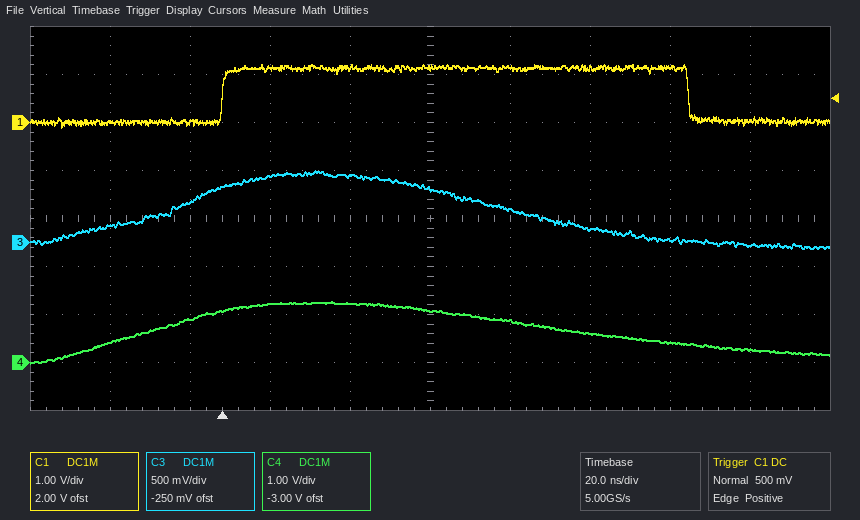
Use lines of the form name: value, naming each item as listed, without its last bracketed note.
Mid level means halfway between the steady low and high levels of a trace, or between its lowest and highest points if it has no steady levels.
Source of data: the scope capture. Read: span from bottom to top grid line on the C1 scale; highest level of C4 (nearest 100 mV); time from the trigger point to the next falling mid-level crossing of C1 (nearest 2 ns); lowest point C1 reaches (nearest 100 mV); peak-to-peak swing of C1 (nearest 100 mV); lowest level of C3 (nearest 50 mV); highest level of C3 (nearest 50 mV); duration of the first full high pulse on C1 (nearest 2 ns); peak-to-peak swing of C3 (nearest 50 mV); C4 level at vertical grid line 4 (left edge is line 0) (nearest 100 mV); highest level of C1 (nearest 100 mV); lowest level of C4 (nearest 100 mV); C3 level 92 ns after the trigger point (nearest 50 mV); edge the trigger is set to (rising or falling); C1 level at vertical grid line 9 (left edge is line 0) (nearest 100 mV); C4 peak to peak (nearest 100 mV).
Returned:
span from bottom to top grid line on the C1 scale: 8 V
highest level of C4: 1.3 V
time from the trigger point to the next falling mid-level crossing of C1: 116 ns
lowest point C1 reaches: -100 mV
peak-to-peak swing of C1: 1.3 V
lowest level of C3: -50 mV
highest level of C3: 750 mV
duration of the first full high pulse on C1: 116 ns
peak-to-peak swing of C3: 800 mV
C4 level at vertical grid line 4 (left edge is line 0): 1.2 V
highest level of C1: 1.2 V
lowest level of C4: 0.0 V
C3 level 92 ns after the trigger point: 150 mV
edge the trigger is set to: rising
C1 level at vertical grid line 9 (left edge is line 0): 0.0 V
C4 peak to peak: 1.3 V
